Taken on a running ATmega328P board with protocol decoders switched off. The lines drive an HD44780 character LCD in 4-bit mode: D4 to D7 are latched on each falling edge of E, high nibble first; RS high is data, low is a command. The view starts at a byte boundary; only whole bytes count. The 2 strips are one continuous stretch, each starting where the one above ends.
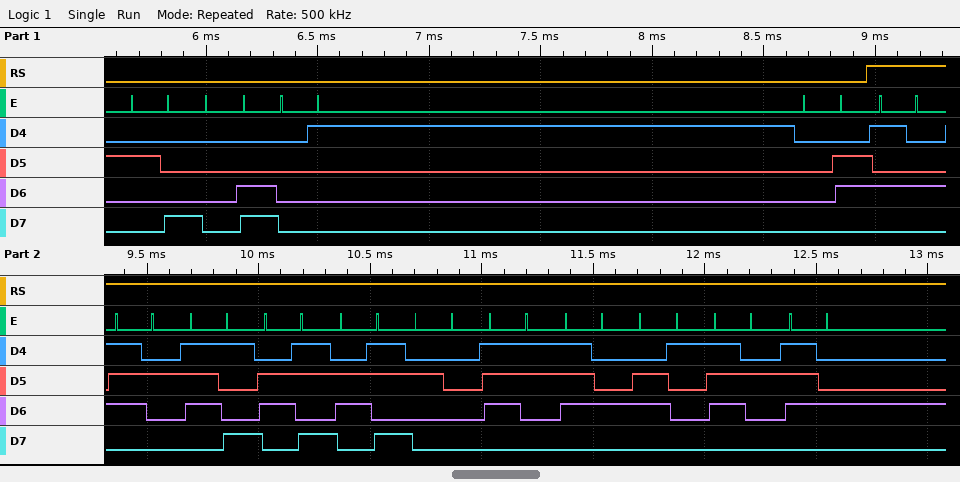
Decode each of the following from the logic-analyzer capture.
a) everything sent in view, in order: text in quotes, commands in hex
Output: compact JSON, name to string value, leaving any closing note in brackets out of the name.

{"everything sent in view, in order: text in quotes, commands in hex": "0x28 0x0C 0x01 0x06 \"Trykk start\""}
